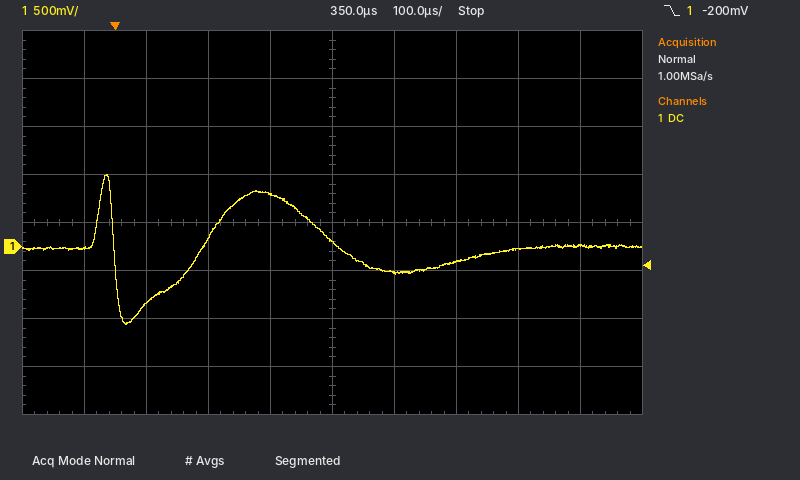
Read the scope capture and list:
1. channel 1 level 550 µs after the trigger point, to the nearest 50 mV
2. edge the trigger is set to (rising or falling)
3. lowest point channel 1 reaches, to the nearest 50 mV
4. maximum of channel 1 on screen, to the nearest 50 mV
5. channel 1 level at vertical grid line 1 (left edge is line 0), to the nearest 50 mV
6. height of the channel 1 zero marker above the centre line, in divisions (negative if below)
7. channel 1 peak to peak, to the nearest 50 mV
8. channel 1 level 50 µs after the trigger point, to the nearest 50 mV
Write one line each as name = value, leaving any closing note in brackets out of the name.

channel 1 level 550 µs after the trigger point, to the nearest 50 mV = -150 mV
edge the trigger is set to = falling
lowest point channel 1 reaches, to the nearest 50 mV = -800 mV
maximum of channel 1 on screen, to the nearest 50 mV = 750 mV
channel 1 level at vertical grid line 1 (left edge is line 0), to the nearest 50 mV = 0 mV
height of the channel 1 zero marker above the centre line, in divisions = -0.5 div
channel 1 peak to peak, to the nearest 50 mV = 1.55 V
channel 1 level 50 µs after the trigger point, to the nearest 50 mV = -600 mV
